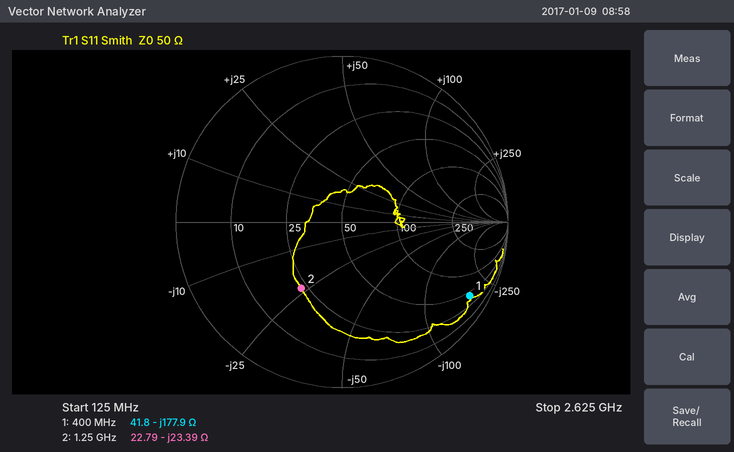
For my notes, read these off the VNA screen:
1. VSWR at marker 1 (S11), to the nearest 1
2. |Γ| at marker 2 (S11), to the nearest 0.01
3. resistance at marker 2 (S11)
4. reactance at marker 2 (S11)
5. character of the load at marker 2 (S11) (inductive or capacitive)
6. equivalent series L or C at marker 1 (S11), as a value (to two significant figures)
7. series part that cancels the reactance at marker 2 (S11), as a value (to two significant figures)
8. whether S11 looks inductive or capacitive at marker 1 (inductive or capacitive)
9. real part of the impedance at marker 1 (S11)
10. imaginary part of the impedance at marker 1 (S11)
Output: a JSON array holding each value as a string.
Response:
["17", "0.47", "22.79 Ω", "-23.39 Ω", "capacitive", "2.2 pF", "3.0 nH", "capacitive", "41.8 Ω", "-177.9 Ω"]
